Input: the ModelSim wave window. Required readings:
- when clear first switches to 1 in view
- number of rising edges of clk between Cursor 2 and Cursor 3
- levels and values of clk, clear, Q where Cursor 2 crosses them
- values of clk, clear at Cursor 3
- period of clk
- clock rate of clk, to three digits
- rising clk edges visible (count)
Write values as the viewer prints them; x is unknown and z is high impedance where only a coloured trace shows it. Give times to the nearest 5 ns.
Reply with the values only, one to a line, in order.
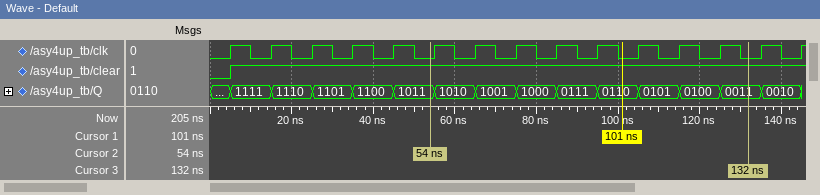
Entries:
5 ns
8
clk=0, clear=1, Q=1011
clk=0, clear=1
10 ns
100 MHz
15
